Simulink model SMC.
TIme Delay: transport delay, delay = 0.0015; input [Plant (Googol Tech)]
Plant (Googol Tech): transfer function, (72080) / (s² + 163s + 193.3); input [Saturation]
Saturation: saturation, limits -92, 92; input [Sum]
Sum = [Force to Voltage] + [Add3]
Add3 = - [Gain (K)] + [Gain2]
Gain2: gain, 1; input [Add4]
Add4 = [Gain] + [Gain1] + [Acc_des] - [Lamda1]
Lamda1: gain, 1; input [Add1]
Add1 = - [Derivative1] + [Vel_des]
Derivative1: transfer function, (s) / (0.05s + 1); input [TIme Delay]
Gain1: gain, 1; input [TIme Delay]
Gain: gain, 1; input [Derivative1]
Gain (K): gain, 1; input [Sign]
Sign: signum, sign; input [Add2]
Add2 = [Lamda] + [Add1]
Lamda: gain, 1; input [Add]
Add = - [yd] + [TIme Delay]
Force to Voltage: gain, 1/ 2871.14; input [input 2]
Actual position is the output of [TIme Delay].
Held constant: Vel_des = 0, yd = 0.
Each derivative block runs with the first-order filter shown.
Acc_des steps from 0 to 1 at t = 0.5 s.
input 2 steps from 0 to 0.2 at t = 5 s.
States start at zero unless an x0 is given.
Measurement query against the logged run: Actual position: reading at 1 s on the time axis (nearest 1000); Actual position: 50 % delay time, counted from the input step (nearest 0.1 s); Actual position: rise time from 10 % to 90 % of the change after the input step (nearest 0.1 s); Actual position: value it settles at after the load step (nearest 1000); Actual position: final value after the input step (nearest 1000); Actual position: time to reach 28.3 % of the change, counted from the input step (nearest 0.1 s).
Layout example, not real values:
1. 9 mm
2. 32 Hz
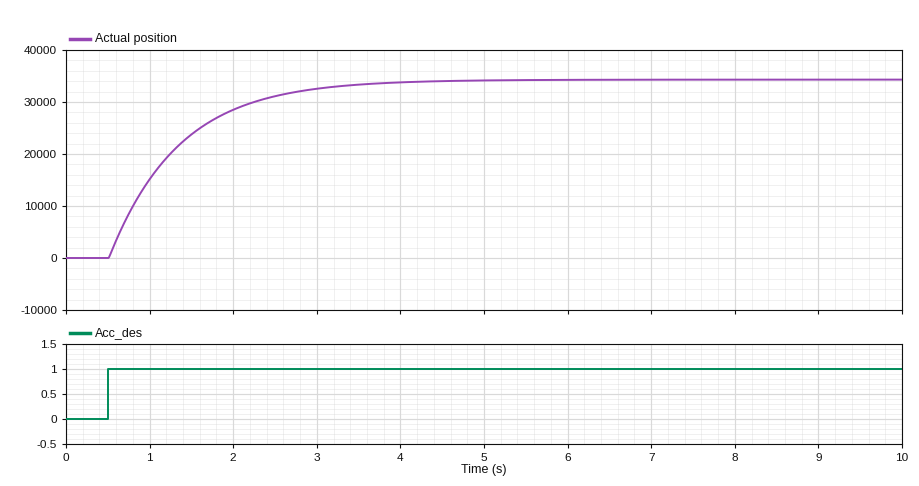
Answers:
1. 15000
2. 0.6 s
3. 1.8 s
4. 34000
5. 34000
6. 0.3 s
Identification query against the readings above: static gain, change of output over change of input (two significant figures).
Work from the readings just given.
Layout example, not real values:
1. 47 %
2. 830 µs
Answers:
1. 34000
